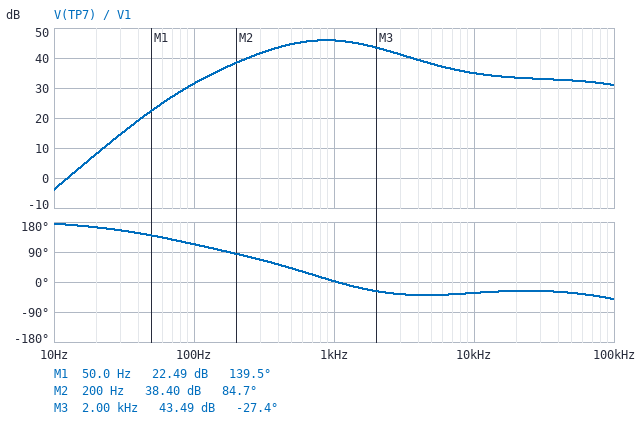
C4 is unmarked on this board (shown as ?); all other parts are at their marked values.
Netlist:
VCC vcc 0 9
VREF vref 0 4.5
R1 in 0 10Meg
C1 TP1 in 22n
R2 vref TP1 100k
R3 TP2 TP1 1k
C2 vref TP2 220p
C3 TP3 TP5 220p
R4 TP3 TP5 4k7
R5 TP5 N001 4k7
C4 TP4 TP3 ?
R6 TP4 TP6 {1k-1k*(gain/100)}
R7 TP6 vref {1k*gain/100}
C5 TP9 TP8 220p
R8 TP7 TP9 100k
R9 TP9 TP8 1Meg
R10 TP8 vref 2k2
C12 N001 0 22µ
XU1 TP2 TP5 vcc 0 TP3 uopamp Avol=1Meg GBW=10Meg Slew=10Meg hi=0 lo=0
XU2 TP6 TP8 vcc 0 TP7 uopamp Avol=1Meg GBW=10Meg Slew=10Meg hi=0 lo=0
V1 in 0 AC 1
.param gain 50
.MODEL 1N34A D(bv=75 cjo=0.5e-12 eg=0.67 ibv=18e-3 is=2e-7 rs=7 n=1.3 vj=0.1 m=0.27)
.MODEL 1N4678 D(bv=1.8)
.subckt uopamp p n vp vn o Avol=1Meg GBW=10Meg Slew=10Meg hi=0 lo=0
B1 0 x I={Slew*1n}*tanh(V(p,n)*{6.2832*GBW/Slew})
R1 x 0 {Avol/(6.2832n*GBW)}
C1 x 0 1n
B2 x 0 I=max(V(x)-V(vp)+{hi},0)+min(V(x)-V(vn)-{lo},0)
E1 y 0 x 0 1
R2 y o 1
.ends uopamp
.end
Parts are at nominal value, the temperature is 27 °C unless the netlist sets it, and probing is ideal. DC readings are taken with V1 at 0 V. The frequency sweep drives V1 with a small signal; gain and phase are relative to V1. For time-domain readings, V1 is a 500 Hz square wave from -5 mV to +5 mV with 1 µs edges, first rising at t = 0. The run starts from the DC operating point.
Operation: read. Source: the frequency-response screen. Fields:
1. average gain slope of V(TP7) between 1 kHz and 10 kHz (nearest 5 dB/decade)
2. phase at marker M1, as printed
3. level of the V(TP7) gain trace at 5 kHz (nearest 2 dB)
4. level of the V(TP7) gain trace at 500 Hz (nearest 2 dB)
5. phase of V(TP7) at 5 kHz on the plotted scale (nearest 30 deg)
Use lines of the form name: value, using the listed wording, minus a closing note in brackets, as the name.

average gain slope of V(TP7) between 1 kHz and 10 kHz: -10 dB/decade
phase at marker M1, as printed: 139.5 deg
level of the V(TP7) gain trace at 5 kHz: 38 dB
level of the V(TP7) gain trace at 500 Hz: 44 dB
phase of V(TP7) at 5 kHz on the plotted scale: -30 deg
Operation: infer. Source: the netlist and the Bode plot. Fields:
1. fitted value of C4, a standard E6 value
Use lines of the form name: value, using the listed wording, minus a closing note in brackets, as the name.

fitted value of C4, a standard E6 value: 150 nF
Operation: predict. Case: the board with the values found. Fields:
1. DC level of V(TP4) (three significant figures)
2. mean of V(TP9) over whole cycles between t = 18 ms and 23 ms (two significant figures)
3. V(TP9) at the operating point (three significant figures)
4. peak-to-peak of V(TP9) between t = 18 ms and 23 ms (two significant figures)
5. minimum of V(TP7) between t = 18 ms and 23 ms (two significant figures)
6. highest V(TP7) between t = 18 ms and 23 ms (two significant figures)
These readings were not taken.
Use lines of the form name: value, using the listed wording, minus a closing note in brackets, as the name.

DC level of V(TP4): 4.50 V
mean of V(TP9) over whole cycles between t = 18 ms and 23 ms: 4.5 V
V(TP9) at the operating point: 4.50 V
peak-to-peak of V(TP9) between t = 18 ms and 23 ms: 2.7 V
minimum of V(TP7) between t = 18 ms and 23 ms: 3.0 V
highest V(TP7) between t = 18 ms and 23 ms: 6.0 V
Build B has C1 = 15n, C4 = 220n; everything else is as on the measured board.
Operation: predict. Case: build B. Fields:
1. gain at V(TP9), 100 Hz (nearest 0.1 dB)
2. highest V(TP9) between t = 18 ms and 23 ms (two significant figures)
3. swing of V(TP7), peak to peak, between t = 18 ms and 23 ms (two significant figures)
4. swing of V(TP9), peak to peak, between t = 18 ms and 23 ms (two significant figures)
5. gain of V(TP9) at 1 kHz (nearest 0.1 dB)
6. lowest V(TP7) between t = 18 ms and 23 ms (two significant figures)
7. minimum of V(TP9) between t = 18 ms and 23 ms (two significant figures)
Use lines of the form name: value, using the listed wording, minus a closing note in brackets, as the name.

gain at V(TP9), 100 Hz: 32.5 dB
highest V(TP9) between t = 18 ms and 23 ms: 6.1 V
swing of V(TP7), peak to peak, between t = 18 ms and 23 ms: 3.6 V
swing of V(TP9), peak to peak, between t = 18 ms and 23 ms: 3.2 V
gain of V(TP9) at 1 kHz: 46.3 dB
lowest V(TP7) between t = 18 ms and 23 ms: 2.7 V
minimum of V(TP9) between t = 18 ms and 23 ms: 2.9 V
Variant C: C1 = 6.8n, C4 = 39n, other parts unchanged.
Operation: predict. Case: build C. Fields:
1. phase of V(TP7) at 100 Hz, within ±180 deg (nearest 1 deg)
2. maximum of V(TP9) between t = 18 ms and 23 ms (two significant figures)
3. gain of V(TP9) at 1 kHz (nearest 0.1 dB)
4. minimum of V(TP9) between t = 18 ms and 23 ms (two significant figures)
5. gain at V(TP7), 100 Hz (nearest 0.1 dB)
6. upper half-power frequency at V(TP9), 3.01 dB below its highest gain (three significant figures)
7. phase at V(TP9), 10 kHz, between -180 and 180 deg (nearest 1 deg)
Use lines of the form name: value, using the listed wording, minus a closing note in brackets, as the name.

phase of V(TP7) at 100 Hz, within ±180 deg: 148 deg
maximum of V(TP9) between t = 18 ms and 23 ms: 5.0 V
gain of V(TP9) at 1 kHz: 35.4 dB
minimum of V(TP9) between t = 18 ms and 23 ms: 4.0 V
gain at V(TP7), 100 Hz: 13.5 dB
upper half-power frequency at V(TP9), 3.01 dB below its highest gain: 5.38 kHz
phase at V(TP9), 10 kHz, between -180 and 180 deg: -66 deg
